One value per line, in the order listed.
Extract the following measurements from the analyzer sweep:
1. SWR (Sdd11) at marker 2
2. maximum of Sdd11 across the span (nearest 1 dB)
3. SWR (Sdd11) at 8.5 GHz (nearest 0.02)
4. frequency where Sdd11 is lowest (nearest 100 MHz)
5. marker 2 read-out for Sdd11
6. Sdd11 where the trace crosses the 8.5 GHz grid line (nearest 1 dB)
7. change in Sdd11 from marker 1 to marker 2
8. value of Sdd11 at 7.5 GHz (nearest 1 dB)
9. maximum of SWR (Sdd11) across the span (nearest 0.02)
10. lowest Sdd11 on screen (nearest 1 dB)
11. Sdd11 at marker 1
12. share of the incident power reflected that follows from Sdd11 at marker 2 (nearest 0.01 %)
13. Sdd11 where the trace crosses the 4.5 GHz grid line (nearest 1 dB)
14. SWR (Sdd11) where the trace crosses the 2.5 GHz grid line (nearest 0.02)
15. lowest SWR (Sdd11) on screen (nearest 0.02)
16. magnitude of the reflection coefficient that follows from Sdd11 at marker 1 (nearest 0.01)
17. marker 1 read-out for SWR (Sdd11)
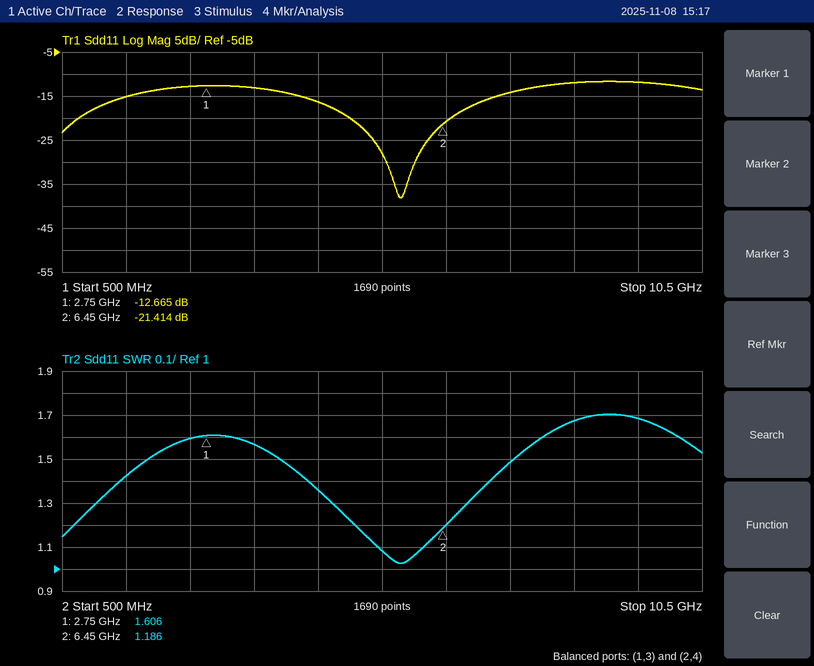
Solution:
1.186
-12 dB
1.68
5.8 GHz
-21.414 dB
-12 dB
-8.749 dB
-14 dB
1.70
-38 dB
-12.665 dB
0.72 %
-16 dB
1.60
1.02
0.23
1.606
